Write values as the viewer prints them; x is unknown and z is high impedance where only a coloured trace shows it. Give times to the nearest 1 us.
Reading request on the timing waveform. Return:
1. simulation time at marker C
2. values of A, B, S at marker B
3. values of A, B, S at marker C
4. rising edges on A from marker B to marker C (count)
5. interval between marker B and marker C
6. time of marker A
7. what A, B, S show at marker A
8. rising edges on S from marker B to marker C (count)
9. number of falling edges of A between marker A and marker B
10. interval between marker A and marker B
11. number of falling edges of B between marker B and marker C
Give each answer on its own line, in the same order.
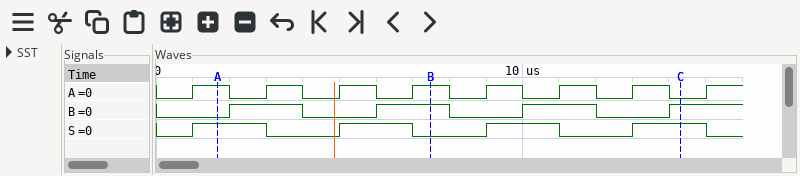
14 us
A=1, B=1, S=0
A=0, B=1, S=1
3
7 us
2 us
A=1, B=0, S=1
2
3
6 us
2
